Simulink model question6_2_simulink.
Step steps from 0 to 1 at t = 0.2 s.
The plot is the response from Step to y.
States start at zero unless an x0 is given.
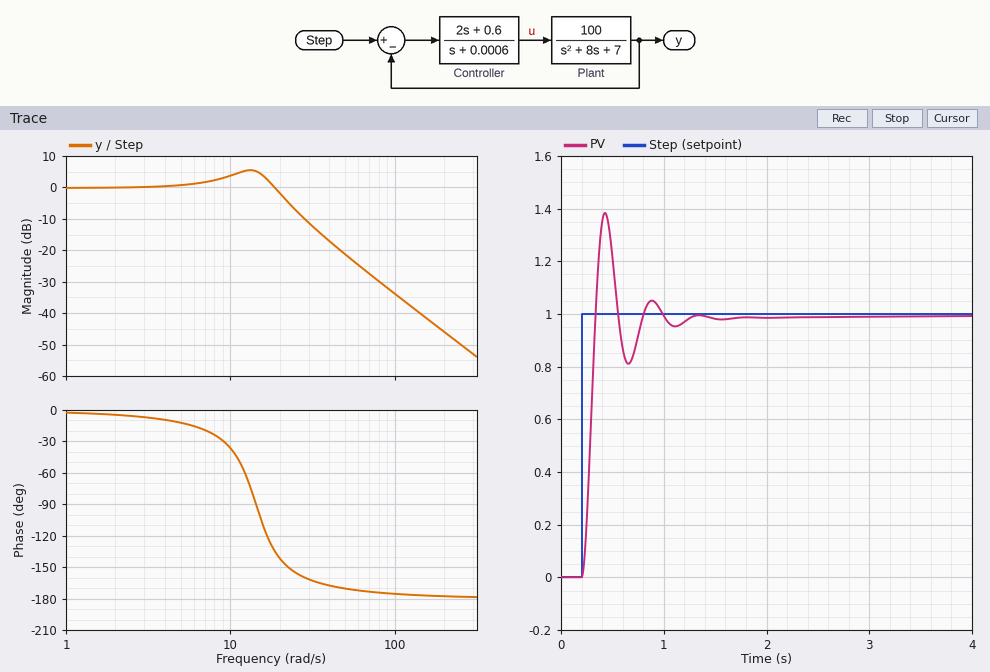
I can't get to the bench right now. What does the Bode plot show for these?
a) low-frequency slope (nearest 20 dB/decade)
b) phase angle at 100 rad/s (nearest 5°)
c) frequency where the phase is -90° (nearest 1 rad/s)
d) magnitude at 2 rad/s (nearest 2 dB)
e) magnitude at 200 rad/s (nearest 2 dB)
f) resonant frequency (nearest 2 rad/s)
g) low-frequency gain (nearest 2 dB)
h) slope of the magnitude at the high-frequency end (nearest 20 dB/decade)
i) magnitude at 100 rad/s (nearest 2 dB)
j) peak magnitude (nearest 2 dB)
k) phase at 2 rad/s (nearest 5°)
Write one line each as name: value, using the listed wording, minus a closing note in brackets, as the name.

low-frequency slope: 0 dB/decade
phase angle at 100 rad/s: -175°
frequency where the phase is -90°: 14 rad/s
magnitude at 2 rad/s: 0 dB
magnitude at 200 rad/s: -46 dB
resonant frequency: 14 rad/s
low-frequency gain: 0 dB
slope of the magnitude at the high-frequency end: -40 dB/decade
magnitude at 100 rad/s: -34 dB
peak magnitude: 6 dB
phase at 2 rad/s: -5°
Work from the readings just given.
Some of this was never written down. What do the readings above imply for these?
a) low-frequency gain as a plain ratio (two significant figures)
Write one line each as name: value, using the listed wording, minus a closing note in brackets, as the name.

low-frequency gain as a plain ratio: 1.0
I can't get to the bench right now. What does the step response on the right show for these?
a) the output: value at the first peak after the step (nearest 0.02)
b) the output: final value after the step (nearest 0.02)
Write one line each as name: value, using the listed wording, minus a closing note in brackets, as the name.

the output: value at the first peak after the step: 1.38
the output: final value after the step: 1.00
